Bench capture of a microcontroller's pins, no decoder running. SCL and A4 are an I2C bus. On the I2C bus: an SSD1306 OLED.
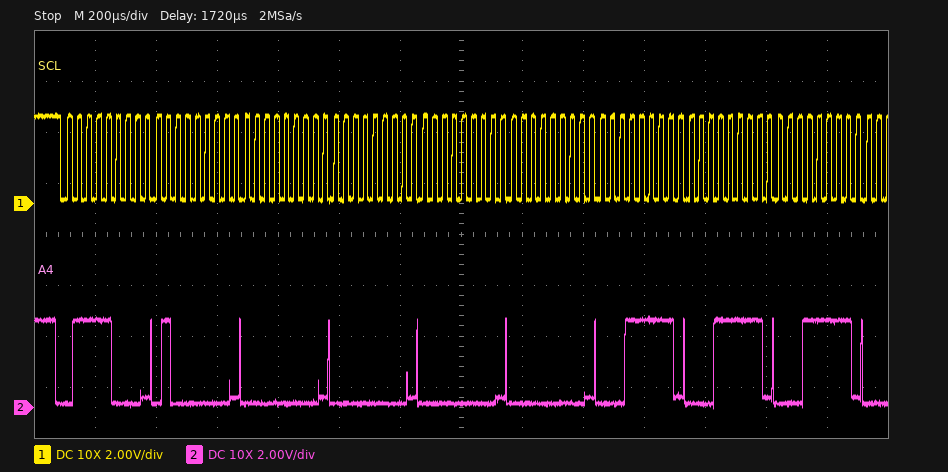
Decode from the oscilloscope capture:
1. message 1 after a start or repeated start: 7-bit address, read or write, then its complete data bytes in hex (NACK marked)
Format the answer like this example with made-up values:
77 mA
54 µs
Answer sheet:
0x3C write: 40 00 00 00 00 1F 1F 1F
